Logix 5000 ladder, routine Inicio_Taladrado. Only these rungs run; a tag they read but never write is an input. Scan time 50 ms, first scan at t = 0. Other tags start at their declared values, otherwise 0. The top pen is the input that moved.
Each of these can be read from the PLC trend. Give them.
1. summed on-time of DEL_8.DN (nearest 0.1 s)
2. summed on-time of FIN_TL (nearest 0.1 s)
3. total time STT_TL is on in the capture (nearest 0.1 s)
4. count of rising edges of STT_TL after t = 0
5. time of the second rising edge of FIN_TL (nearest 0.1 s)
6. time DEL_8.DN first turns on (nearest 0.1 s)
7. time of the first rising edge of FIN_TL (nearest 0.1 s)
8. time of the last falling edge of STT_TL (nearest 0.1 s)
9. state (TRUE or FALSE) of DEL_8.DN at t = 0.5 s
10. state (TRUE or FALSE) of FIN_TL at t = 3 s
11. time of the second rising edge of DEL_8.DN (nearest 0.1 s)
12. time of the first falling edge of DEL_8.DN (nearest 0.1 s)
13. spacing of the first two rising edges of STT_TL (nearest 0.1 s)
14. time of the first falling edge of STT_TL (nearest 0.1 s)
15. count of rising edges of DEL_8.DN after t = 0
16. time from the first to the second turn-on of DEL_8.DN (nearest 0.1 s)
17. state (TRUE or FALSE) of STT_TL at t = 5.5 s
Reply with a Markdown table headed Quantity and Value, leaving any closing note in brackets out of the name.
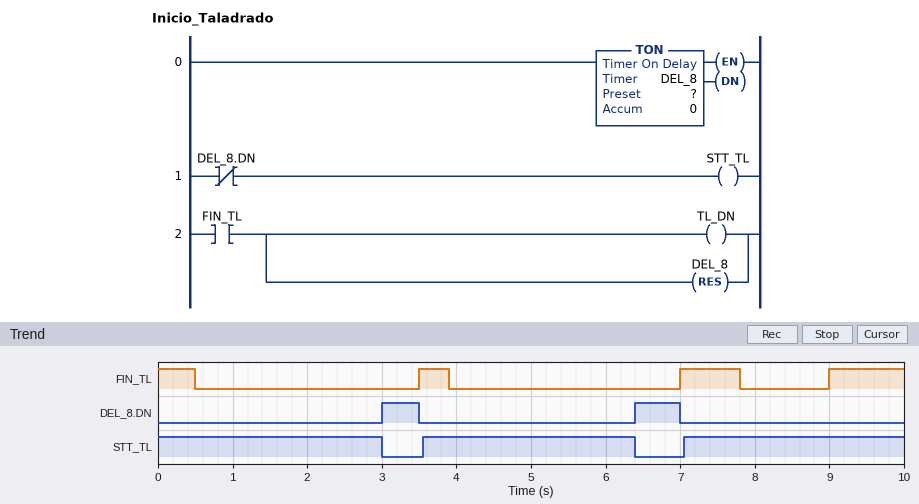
| Quantity | Value |
|---|---|
| summed on-time of DEL_8.DN | 1.1 s |
| summed on-time of FIN_TL | 2.7 s |
| total time STT_TL is on in the capture | 8.8 s |
| count of rising edges of STT_TL after t = 0 | 2 |
| time of the second rising edge of FIN_TL | 7.0 s |
| time DEL_8.DN first turns on | 3.0 s |
| time of the first rising edge of FIN_TL | 3.5 s |
| time of the last falling edge of STT_TL | 6.4 s |
| state (TRUE or FALSE) of DEL_8.DN at t = 0.5 s | FALSE |
| state (TRUE or FALSE) of FIN_TL at t = 3 s | FALSE |
| time of the second rising edge of DEL_8.DN | 6.4 s |
| time of the first falling edge of DEL_8.DN | 3.5 s |
| spacing of the first two rising edges of STT_TL | 3.5 s |
| time of the first falling edge of STT_TL | 3.0 s |
| count of rising edges of DEL_8.DN after t = 0 | 2 |
| time from the first to the second turn-on of DEL_8.DN | 3.4 s |
| state (TRUE or FALSE) of STT_TL at t = 5.5 s | TRUE |
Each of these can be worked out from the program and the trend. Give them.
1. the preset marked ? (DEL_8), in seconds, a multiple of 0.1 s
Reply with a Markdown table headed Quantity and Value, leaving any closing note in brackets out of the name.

| Quantity | Value |
|---|---|
| the preset marked ? (DEL_8), in seconds, a multiple of 0.1 s | 2.5 s |
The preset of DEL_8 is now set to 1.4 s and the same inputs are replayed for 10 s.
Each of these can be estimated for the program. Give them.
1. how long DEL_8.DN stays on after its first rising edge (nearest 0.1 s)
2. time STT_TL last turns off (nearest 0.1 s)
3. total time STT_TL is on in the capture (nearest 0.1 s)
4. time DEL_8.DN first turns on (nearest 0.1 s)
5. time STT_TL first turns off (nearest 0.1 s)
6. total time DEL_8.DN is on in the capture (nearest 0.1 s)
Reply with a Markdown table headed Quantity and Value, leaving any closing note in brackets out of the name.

| Quantity | Value |
|---|---|
| how long DEL_8.DN stays on after its first rising edge | 1.6 s |
| time STT_TL last turns off | 5.3 s |
| total time STT_TL is on in the capture | 6.6 s |
| time DEL_8.DN first turns on | 1.9 s |
| time STT_TL first turns off | 1.9 s |
| total time DEL_8.DN is on in the capture | 3.3 s |
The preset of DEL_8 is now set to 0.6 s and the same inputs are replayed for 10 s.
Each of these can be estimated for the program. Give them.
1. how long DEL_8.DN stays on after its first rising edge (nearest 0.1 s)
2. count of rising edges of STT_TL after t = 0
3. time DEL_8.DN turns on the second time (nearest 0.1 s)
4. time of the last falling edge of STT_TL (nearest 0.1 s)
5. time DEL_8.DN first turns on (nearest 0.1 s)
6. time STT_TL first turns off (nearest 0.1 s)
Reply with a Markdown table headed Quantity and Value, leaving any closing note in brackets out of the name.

| Quantity | Value |
|---|---|
| how long DEL_8.DN stays on after its first rising edge | 2.4 s |
| count of rising edges of STT_TL after t = 0 | 3 |
| time DEL_8.DN turns on the second time | 4.5 s |
| time of the last falling edge of STT_TL | 8.4 s |
| time DEL_8.DN first turns on | 1.1 s |
| time STT_TL first turns off | 1.1 s |
